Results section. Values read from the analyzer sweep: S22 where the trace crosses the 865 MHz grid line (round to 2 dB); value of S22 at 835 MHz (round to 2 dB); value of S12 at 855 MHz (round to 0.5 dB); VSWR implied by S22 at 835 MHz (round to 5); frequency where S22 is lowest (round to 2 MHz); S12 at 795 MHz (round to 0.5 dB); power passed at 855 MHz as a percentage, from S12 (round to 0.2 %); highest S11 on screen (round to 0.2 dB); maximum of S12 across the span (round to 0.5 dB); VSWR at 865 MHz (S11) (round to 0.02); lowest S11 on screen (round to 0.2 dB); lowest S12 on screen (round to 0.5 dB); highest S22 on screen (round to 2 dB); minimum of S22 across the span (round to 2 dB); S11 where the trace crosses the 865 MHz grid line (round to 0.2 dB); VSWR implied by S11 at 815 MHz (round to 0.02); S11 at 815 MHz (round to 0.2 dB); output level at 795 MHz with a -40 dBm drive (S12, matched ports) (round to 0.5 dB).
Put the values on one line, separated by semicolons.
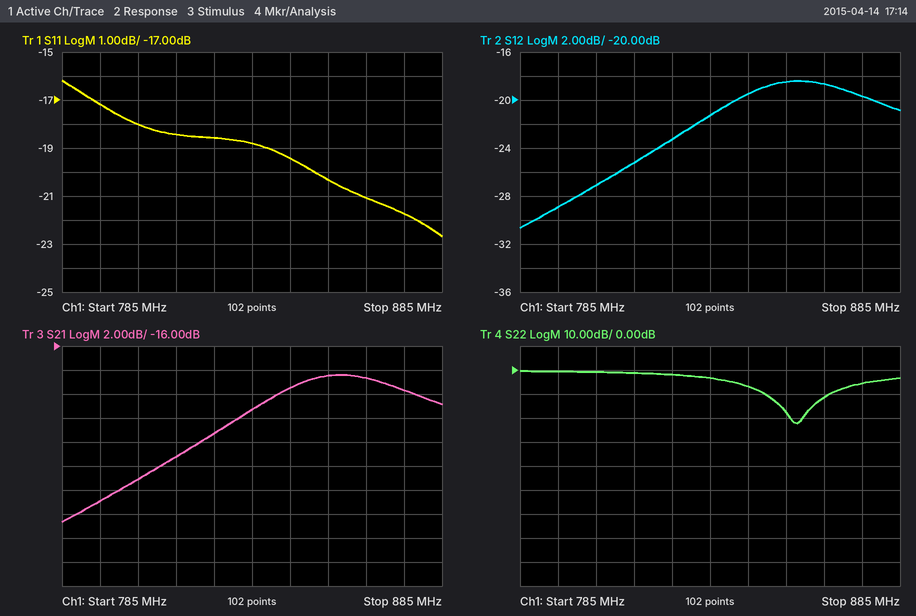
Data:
-12 dB; -4 dB; -18.5 dB; 5; 858 MHz; -29.0 dB; 1.4 %; -16.2 dB; -18.5 dB; 1.20; -22.6 dB; -30.5 dB; 0 dB; -22 dB; -21.0 dB; 1.28; -18.4 dB; -69.0 dBm
